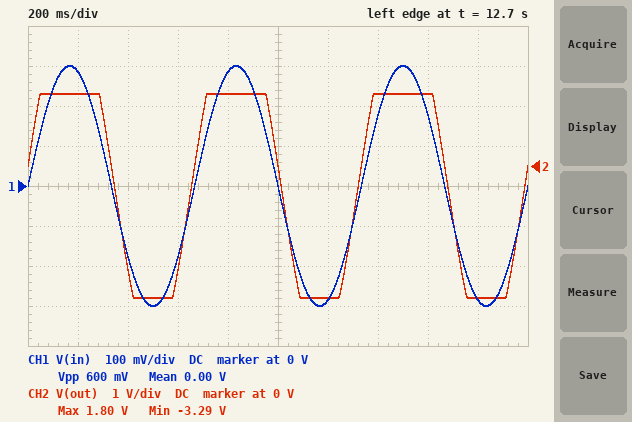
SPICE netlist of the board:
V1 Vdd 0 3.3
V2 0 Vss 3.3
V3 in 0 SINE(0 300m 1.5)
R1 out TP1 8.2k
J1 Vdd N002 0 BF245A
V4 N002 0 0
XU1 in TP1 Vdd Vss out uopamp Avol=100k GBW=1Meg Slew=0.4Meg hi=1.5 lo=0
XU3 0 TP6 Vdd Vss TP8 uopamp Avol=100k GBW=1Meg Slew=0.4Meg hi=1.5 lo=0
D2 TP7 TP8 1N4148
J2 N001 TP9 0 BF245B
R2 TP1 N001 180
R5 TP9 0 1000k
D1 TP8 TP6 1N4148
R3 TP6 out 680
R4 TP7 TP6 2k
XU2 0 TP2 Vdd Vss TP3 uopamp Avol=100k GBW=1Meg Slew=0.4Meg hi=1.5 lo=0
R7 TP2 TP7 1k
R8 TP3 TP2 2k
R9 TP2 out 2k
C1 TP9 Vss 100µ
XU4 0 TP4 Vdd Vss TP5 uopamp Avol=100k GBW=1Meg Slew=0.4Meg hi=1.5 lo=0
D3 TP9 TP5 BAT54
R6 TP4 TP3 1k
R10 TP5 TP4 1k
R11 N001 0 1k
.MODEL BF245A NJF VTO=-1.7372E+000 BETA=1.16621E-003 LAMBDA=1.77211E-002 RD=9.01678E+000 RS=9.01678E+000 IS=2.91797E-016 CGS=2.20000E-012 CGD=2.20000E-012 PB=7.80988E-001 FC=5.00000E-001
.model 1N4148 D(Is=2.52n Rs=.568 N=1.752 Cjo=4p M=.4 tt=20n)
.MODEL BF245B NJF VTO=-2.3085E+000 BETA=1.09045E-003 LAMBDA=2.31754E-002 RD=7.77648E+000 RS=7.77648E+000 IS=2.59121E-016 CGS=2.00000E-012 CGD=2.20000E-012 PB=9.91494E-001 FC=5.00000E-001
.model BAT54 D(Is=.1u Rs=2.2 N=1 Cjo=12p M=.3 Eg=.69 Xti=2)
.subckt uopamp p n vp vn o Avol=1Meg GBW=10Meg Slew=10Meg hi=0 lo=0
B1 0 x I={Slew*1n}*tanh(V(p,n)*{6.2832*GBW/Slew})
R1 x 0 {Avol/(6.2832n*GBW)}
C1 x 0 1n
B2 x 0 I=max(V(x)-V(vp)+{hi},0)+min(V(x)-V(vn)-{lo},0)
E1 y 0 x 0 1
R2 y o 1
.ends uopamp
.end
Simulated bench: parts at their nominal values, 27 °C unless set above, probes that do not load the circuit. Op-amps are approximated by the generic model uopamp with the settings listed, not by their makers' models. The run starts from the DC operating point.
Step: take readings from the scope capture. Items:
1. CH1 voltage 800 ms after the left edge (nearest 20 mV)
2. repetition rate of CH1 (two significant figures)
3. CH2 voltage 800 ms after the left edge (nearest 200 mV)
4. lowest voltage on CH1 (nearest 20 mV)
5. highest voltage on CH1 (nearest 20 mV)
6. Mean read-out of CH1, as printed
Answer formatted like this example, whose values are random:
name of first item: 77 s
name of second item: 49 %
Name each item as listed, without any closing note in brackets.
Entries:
CH1 voltage 800 ms after the left edge: 280 mV
repetition rate of CH1: 1.5 Hz
CH2 voltage 800 ms after the left edge: 1.8 V
lowest voltage on CH1: -300 mV
highest voltage on CH1: 300 mV
Mean read-out of CH1, as printed: 0.00 V
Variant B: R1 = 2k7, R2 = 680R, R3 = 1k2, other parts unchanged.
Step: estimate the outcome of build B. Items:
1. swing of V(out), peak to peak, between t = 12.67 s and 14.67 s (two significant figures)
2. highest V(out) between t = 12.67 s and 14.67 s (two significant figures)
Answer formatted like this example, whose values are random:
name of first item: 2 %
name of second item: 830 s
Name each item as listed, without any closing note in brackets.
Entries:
swing of V(out), peak to peak, between t = 12.67 s and 14.67 s: 2.1 V
highest V(out) between t = 12.67 s and 14.67 s: 1.0 V
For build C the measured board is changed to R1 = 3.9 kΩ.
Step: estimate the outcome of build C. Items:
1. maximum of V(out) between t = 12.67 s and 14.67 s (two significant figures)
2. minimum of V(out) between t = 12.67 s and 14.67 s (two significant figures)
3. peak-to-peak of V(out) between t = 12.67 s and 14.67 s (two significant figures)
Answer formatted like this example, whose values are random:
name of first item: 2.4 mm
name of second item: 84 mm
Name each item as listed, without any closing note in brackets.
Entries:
maximum of V(out) between t = 12.67 s and 14.67 s: 1.8 V
minimum of V(out) between t = 12.67 s and 14.67 s: -2.3 V
peak-to-peak of V(out) between t = 12.67 s and 14.67 s: 4.1 V
